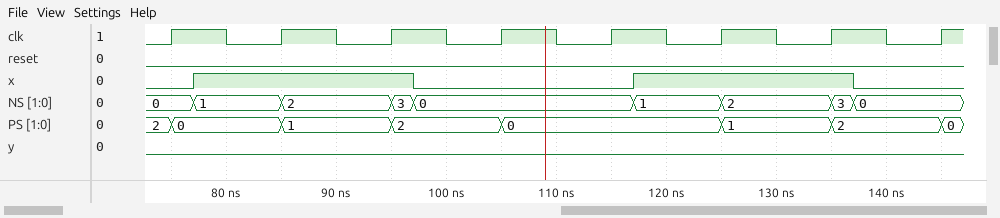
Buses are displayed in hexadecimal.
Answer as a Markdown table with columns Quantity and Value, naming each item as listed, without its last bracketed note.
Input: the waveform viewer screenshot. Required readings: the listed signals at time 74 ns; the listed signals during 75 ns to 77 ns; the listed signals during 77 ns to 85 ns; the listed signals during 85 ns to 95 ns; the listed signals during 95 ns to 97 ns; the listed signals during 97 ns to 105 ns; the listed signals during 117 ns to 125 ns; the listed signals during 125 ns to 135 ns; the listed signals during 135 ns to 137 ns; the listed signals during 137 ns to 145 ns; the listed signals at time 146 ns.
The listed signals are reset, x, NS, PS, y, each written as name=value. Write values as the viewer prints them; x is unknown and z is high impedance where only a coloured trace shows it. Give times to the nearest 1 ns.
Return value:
| Quantity | Value |
|---|---|
| the listed signals at time 74 ns | reset=0, x=0, NS=0, PS=2, y=0 |
| the listed signals during 75 ns to 77 ns | reset=0, x=0, NS=0, PS=0, y=0 |
| the listed signals during 77 ns to 85 ns | reset=0, x=1, NS=1, PS=0, y=0 |
| the listed signals during 85 ns to 95 ns | reset=0, x=1, NS=2, PS=1, y=0 |
| the listed signals during 95 ns to 97 ns | reset=0, x=1, NS=3, PS=2, y=0 |
| the listed signals during 97 ns to 105 ns | reset=0, x=0, NS=0, PS=2, y=0 |
| the listed signals during 117 ns to 125 ns | reset=0, x=1, NS=1, PS=0, y=0 |
| the listed signals during 125 ns to 135 ns | reset=0, x=1, NS=2, PS=1, y=0 |
| the listed signals during 135 ns to 137 ns | reset=0, x=1, NS=3, PS=2, y=0 |
| the listed signals during 137 ns to 145 ns | reset=0, x=0, NS=0, PS=2, y=0 |
| the listed signals at time 146 ns | reset=0, x=0, NS=0, PS=0, y=0 |
